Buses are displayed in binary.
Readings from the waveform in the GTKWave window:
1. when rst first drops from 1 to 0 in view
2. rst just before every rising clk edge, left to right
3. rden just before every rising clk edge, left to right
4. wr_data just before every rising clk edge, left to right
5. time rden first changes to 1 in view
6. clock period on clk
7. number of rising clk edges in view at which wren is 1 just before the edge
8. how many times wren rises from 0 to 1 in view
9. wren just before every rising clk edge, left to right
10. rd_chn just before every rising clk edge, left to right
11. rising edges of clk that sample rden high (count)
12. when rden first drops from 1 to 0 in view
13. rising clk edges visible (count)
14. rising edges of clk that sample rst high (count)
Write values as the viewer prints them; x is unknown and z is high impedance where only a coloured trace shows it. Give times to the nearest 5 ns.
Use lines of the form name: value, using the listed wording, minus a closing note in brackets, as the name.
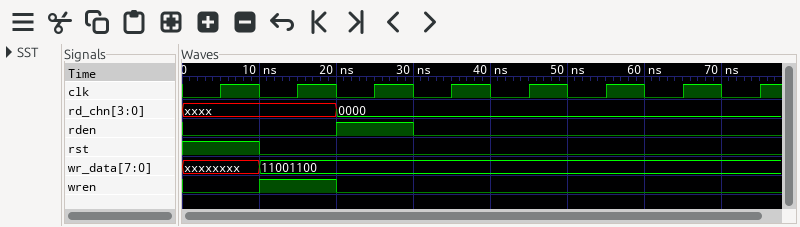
when rst first drops from 1 to 0 in view: 10 ns
rst just before every rising clk edge, left to right: 1 0 0 0 0 0 0 0
rden just before every rising clk edge, left to right: 0 0 1 0 0 0 0 0
wr_data just before every rising clk edge, left to right: xxxxxxxx, 11001100, 11001100, 11001100, 11001100, 11001100, 11001100, 11001100
time rden first changes to 1 in view: 20 ns
clock period on clk: 10 ns
number of rising clk edges in view at which wren is 1 just before the edge: 1
how many times wren rises from 0 to 1 in view: 1
wren just before every rising clk edge, left to right: 0 1 0 0 0 0 0 0
rd_chn just before every rising clk edge, left to right: xxxx, xxxx, 0000, 0000, 0000, 0000, 0000, 0000
rising edges of clk that sample rden high: 1
when rden first drops from 1 to 0 in view: 30 ns
rising clk edges visible: 8
rising edges of clk that sample rst high: 1
